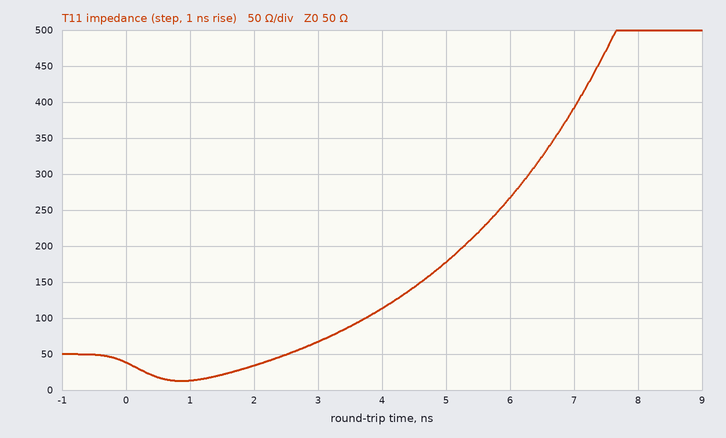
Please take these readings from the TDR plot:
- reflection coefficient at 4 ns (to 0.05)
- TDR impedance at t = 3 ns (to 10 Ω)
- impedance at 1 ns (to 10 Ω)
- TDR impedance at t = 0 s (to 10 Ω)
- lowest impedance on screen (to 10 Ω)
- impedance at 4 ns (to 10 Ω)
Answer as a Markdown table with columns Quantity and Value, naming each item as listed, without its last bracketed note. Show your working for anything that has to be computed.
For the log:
| Quantity | Value |
|---|---|
| reflection coefficient at 4 ns | (110 − 50)/(110 + 50) ≈ +0.375, so +0.40 to the nearest 0.05 |
| TDR impedance at t = 3 ns | 70 Ω |
| impedance at 1 ns | 10 Ω |
| TDR impedance at t = 0 s | 40 Ω |
| lowest impedance on screen | 10 Ω |
| impedance at 4 ns | 110 Ω |
